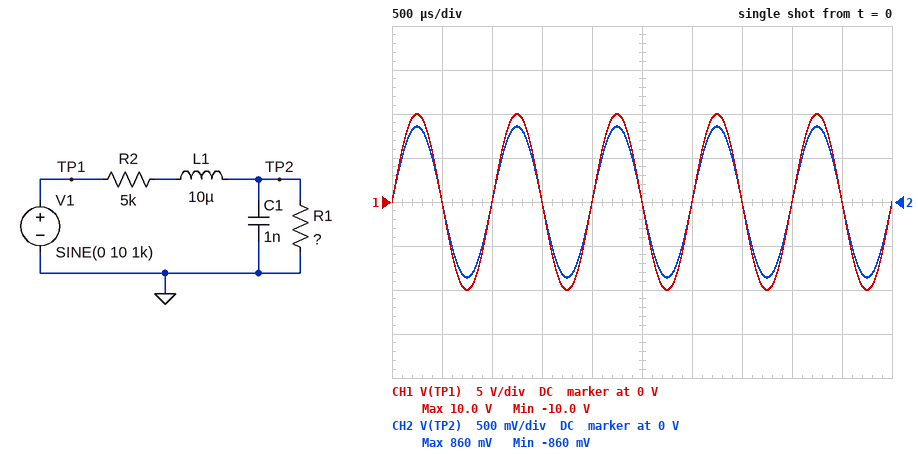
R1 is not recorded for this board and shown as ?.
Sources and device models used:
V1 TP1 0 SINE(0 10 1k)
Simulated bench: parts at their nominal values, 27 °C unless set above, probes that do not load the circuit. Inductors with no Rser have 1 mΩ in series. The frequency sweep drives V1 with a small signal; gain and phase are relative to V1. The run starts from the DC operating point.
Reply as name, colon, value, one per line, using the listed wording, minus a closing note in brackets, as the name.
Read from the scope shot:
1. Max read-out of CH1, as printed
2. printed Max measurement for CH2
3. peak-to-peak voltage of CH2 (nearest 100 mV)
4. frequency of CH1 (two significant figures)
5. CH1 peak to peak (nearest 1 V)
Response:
Max read-out of CH1, as printed: 10.0 V
printed Max measurement for CH2: 860 mV
peak-to-peak voltage of CH2: 1.7 V
frequency of CH1: 1.0 kHz
CH1 peak to peak: 20 V
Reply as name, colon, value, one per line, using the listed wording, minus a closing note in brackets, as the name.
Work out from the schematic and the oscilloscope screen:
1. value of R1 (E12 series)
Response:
value of R1: 470 Ω
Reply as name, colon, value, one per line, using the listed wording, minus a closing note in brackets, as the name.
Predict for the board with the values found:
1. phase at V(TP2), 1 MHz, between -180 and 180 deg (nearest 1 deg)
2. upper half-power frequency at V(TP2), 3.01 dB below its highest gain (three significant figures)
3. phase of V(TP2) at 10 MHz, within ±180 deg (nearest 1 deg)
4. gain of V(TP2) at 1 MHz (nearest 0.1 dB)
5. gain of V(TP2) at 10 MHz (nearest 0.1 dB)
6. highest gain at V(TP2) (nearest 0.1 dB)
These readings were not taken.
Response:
phase at V(TP2), 1 MHz, between -180 and 180 deg: -70 deg
upper half-power frequency at V(TP2), 3.01 dB below its highest gain: 371 kHz
phase of V(TP2) at 10 MHz, within ±180 deg: -95 deg
gain of V(TP2) at 1 MHz: -30.5 dB
gain of V(TP2) at 10 MHz: -50.0 dB
highest gain at V(TP2): -21.3 dB
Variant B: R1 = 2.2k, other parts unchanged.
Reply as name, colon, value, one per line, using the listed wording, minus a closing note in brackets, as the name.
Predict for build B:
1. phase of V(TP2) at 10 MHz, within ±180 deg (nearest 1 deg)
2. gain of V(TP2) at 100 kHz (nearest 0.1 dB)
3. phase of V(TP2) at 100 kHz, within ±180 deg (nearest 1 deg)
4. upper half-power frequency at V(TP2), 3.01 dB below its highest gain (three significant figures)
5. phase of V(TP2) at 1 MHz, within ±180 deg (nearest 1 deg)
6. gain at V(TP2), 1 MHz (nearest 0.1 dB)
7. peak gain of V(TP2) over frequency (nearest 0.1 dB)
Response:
phase of V(TP2) at 10 MHz, within ±180 deg: -97 deg
gain of V(TP2) at 100 kHz: -13.1 dB
phase of V(TP2) at 100 kHz, within ±180 deg: -44 deg
upper half-power frequency at V(TP2), 3.01 dB below its highest gain: 104 kHz
phase of V(TP2) at 1 MHz, within ±180 deg: -85 deg
gain at V(TP2), 1 MHz: -30.0 dB
peak gain of V(TP2) over frequency: -10.3 dB
